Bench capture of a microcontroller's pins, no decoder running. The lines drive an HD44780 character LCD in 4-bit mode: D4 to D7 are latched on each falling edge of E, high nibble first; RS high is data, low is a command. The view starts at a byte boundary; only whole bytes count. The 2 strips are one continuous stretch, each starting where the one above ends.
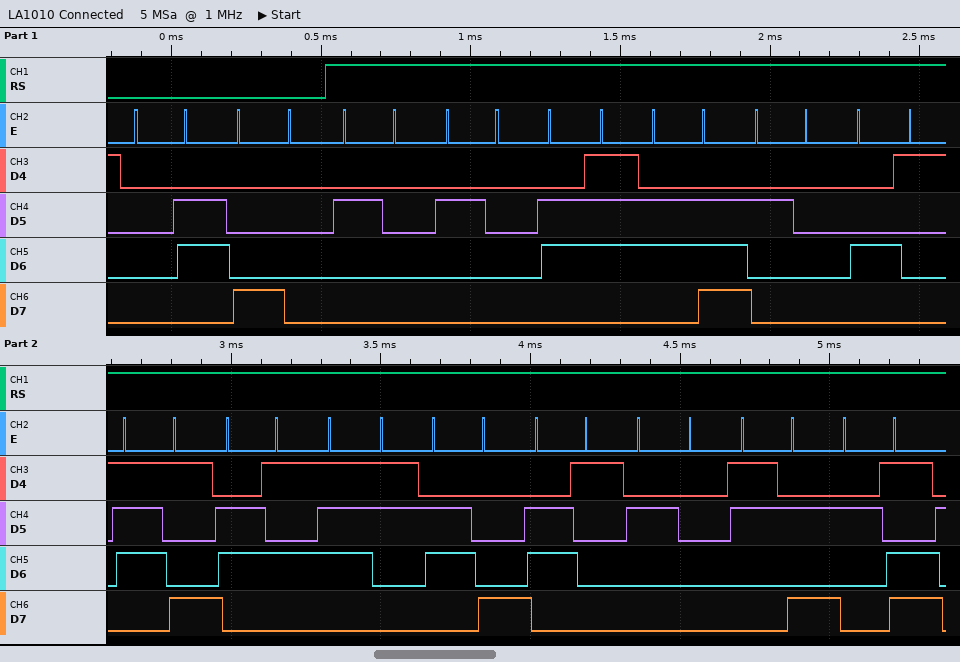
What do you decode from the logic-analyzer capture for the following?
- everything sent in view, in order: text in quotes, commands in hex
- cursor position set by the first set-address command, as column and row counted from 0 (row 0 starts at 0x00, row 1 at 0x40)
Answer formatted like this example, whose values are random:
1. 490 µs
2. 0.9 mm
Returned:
1. 0x06 0x80 "  gn Ayesha :-"
2. column 0, row 0
